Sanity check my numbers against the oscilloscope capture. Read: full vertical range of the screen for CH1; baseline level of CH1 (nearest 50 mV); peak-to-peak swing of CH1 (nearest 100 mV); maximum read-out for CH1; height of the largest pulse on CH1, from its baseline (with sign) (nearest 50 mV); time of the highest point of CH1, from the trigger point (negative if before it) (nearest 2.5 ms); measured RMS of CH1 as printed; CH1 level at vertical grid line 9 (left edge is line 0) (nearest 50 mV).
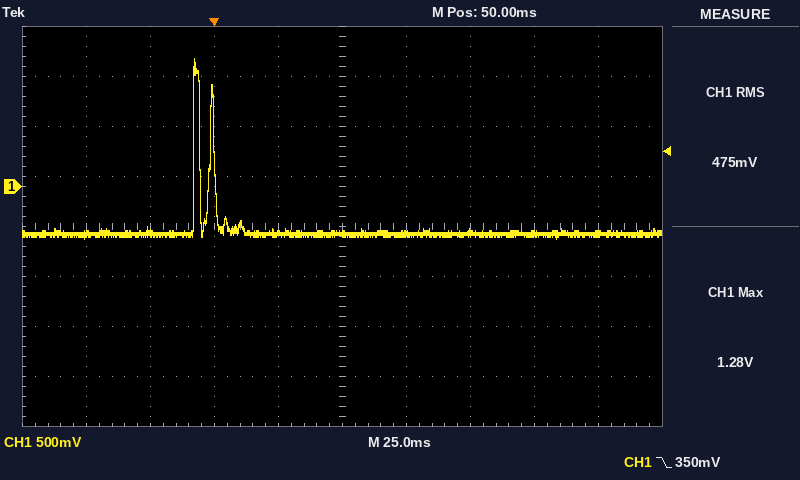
4 V
-450 mV
1.80 V
1.28 V
+1.75 V
-7.5 ms
475 mV
-450 mV
